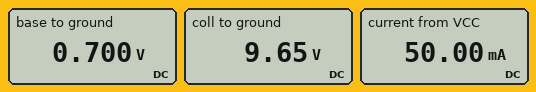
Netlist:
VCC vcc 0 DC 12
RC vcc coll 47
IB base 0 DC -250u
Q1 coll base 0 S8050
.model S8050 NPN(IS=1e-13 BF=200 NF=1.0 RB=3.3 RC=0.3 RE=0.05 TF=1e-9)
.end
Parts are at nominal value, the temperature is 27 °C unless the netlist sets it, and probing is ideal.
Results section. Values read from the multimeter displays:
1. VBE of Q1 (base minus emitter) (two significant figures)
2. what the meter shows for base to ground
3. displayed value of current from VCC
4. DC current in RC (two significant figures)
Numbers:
700 mV
0.700 V
50.00 mA
50 mA
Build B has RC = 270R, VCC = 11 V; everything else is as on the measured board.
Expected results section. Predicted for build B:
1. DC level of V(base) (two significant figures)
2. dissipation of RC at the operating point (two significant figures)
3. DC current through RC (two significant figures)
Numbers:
690 mV
430 mW
40 mA
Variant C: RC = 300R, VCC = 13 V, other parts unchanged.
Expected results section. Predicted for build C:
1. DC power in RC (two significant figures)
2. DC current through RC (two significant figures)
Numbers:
550 mW
43 mA
